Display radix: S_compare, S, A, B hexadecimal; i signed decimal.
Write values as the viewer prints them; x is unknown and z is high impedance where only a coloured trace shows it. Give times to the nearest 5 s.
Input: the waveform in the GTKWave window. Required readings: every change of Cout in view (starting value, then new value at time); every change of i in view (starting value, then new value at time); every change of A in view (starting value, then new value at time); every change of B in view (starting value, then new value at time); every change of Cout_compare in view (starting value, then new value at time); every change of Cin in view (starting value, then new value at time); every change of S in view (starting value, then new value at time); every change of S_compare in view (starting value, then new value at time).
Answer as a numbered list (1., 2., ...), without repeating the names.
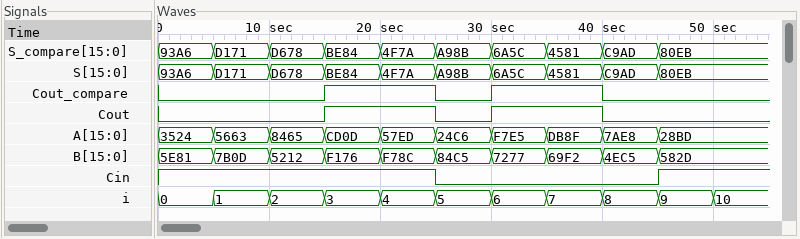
1. 0, 1 at 15 s, 0 at 25 s, 1 at 30 s, 0 at 40 s
2. 0, 1 at 5 s, 2 at 10 s, 3 at 15 s, 4 at 20 s, 5 at 25 s, 6 at 30 s, 7 at 35 s, 8 at 40 s, 9 at 45 s, 10 at 50 s
3. 3524, 5663 at 5 s, 8465 at 10 s, CD0D at 15 s, 57ED at 20 s, 24C6 at 25 s, F7E5 at 30 s, DB8F at 35 s, 7AE8 at 40 s, 28BD at 45 s
4. 5E81, 7B0D at 5 s, 5212 at 10 s, F176 at 15 s, F78C at 20 s, 84C5 at 25 s, 7277 at 30 s, 69F2 at 35 s, 4EC5 at 40 s, 582D at 45 s
5. 0, 1 at 15 s, 0 at 25 s, 1 at 30 s, 0 at 40 s
6. 1, 0 at 25 s, 1 at 45 s
7. 93A6, D171 at 5 s, D678 at 10 s, BE84 at 15 s, 4F7A at 20 s, A98B at 25 s, 6A5C at 30 s, 4581 at 35 s, C9AD at 40 s, 80EB at 45 s
8. 93A6, D171 at 5 s, D678 at 10 s, BE84 at 15 s, 4F7A at 20 s, A98B at 25 s, 6A5C at 30 s, 4581 at 35 s, C9AD at 40 s, 80EB at 45 s
